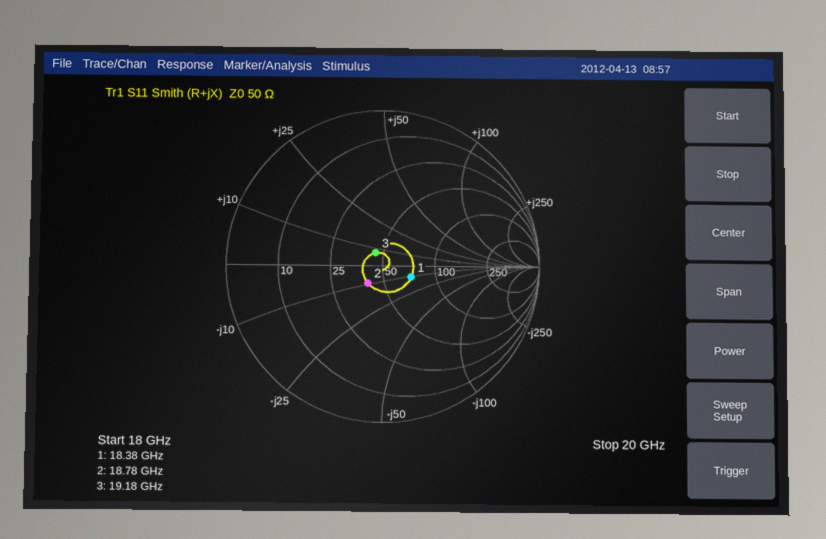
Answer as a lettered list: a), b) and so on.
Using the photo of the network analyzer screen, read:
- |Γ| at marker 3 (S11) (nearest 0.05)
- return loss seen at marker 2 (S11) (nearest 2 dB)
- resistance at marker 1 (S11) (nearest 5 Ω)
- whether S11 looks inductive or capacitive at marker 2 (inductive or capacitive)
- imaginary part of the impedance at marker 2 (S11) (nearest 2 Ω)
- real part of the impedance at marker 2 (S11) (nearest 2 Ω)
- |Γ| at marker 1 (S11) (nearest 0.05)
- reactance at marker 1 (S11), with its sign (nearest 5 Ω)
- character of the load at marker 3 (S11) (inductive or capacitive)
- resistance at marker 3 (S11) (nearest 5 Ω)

a) 0.10
b) 16 dB
c) 70 Ω
d) capacitive
e) -10 Ω
f) 40 Ω
g) 0.20
h) -10 Ω
i) inductive
j) 45 Ω
